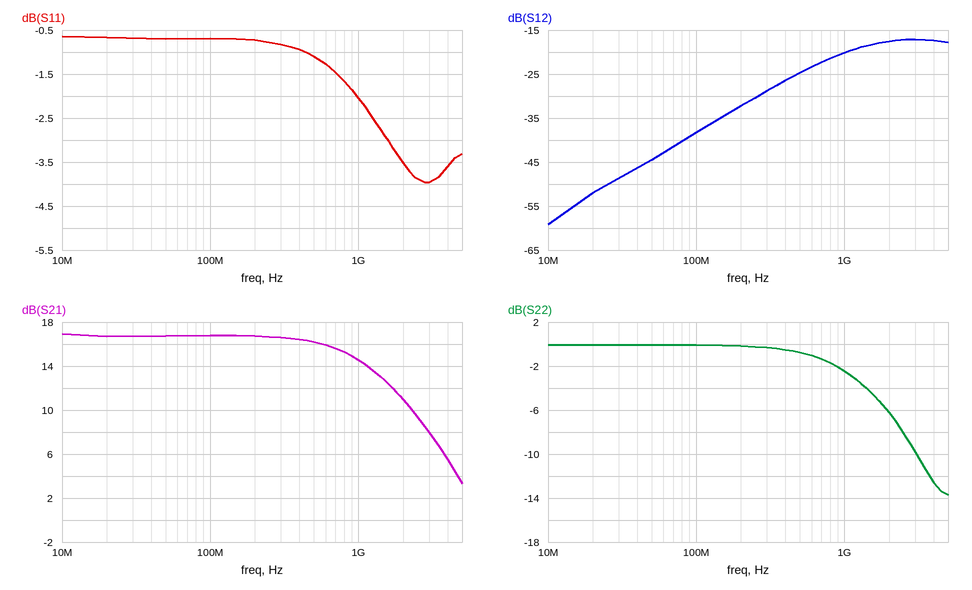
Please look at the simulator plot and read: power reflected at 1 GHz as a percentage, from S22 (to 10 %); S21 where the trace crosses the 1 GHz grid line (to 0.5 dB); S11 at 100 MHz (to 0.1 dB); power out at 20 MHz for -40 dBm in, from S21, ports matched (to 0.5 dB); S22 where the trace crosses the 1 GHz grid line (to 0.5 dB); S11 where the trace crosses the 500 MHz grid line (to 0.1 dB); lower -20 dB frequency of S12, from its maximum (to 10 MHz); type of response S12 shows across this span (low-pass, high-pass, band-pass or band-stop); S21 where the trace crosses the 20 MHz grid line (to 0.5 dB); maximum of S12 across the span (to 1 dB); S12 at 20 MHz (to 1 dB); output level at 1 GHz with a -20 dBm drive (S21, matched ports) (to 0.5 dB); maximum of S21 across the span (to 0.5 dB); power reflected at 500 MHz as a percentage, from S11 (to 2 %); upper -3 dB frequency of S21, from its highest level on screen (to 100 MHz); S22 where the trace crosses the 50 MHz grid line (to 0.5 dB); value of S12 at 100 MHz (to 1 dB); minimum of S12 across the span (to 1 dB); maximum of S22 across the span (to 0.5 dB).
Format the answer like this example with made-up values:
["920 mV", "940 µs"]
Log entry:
["60 %", "14.5 dB", "-0.7 dB", "-23.5 dBm", "-2.5 dB", "-1.1 dB", "110 MHz", "high-pass", "16.5 dB", "-17 dB", "-52 dB", "-5.5 dBm", "17.0 dB", "78 %", "1.2 GHz", "0.0 dB", "-38 dB", "-59 dB", "0.0 dB"]
